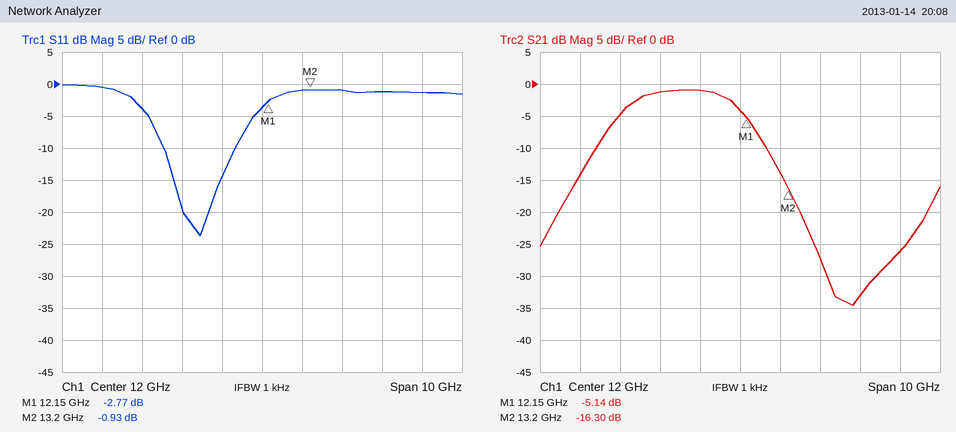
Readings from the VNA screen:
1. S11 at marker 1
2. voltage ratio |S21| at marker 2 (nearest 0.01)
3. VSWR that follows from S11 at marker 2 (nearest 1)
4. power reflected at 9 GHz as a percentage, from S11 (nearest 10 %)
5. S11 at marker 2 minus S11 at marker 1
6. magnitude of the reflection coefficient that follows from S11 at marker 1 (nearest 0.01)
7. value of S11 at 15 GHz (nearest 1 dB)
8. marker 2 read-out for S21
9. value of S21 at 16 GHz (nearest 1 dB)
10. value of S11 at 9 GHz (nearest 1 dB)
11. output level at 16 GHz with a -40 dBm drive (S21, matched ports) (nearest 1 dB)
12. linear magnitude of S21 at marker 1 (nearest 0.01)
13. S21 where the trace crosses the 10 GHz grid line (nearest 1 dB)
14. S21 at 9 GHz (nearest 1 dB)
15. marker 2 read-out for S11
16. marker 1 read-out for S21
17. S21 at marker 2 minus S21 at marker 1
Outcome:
-2.77 dB
0.15
19
40 %
1.84 dB
0.73
-1 dB
-16.30 dB
-26 dB
-4 dB
-66 dBm
0.55
-1 dB
-5 dB
-0.93 dB
-5.14 dB
-11.16 dB
